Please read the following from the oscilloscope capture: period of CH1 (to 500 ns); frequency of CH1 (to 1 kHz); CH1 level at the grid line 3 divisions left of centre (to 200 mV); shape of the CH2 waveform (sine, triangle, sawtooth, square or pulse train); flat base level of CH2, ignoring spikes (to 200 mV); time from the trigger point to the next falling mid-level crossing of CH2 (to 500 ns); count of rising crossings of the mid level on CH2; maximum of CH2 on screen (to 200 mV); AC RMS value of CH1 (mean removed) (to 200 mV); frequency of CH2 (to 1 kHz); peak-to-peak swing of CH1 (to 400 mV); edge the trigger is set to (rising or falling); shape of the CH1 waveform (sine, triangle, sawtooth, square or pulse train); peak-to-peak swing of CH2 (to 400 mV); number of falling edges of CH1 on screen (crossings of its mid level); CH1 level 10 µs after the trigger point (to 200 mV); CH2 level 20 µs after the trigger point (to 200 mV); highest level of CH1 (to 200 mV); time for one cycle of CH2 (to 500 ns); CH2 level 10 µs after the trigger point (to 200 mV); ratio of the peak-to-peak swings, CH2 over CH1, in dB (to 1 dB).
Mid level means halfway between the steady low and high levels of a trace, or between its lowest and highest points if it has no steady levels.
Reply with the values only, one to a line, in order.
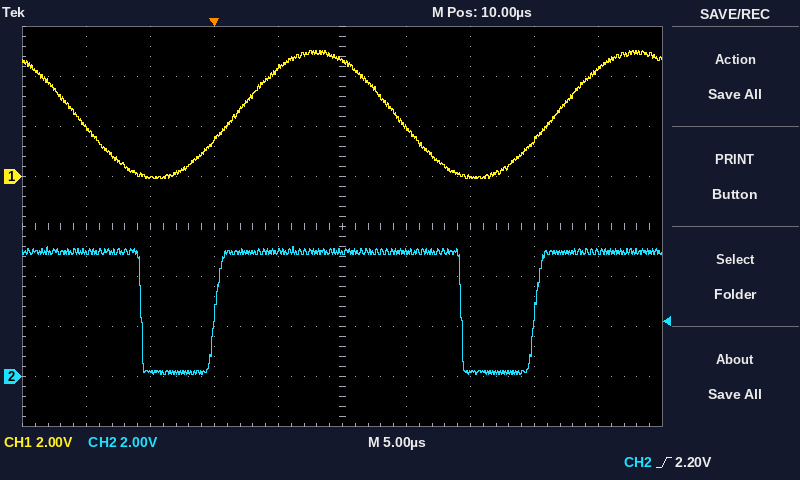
25.0 µs
40 kHz
0.0 V
pulse train
200 mV
19.5 µs
2
5.2 V
1.8 V
40 kHz
5.2 V
rising
sine
5.2 V
2
4.6 V
200 mV
5.0 V
25.0 µs
5.0 V
0 dB
